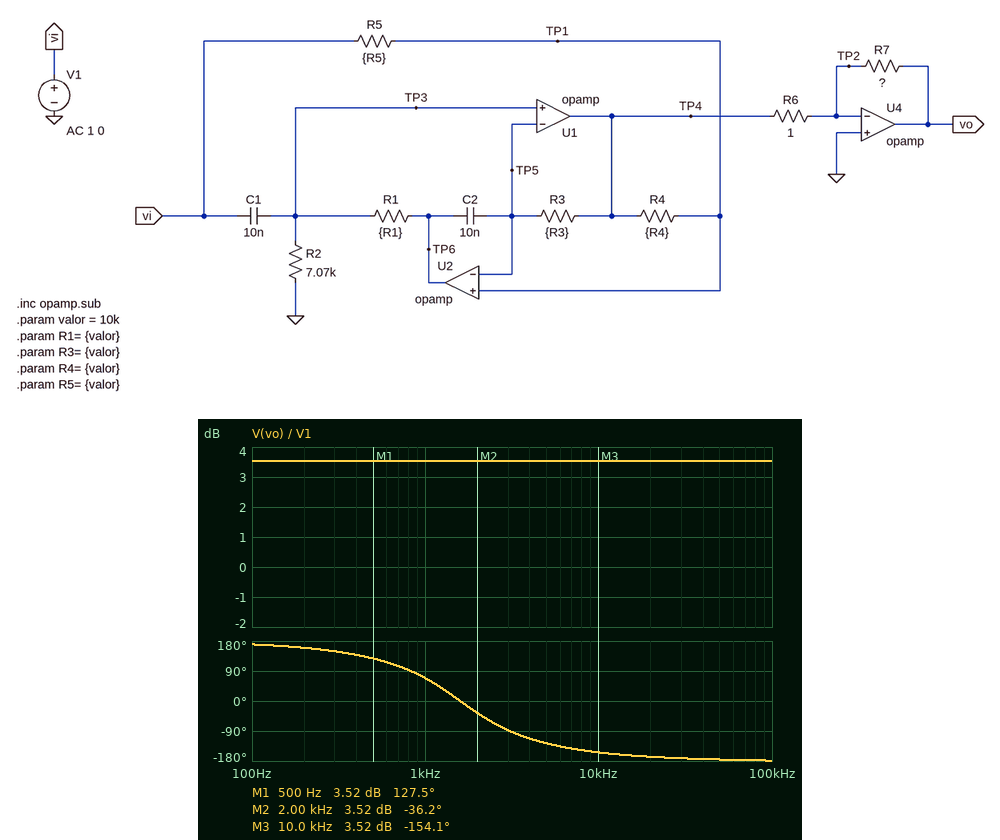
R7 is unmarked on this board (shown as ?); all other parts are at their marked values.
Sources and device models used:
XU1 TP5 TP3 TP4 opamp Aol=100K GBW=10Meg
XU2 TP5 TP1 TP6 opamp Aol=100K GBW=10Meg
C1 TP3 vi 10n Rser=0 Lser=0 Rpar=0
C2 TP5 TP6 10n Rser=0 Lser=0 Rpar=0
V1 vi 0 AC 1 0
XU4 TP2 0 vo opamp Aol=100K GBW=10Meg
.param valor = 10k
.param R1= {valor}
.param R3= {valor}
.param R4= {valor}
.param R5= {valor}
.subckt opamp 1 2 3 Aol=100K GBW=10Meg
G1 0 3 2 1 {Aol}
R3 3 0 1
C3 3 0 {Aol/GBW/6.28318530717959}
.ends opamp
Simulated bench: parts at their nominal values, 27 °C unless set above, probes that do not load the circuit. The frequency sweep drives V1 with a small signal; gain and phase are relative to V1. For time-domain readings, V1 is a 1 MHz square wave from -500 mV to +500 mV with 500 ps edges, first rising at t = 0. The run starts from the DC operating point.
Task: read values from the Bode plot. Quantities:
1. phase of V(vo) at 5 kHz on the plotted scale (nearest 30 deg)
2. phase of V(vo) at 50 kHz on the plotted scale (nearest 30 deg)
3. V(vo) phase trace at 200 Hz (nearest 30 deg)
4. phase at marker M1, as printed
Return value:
-120 deg
-180 deg
150 deg
127.5 deg
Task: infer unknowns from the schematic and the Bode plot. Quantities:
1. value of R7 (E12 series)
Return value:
1.5 Ω
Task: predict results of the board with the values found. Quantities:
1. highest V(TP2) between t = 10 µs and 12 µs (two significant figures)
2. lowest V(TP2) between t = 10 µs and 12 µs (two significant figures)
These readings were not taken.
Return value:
420 mV
-420 mV
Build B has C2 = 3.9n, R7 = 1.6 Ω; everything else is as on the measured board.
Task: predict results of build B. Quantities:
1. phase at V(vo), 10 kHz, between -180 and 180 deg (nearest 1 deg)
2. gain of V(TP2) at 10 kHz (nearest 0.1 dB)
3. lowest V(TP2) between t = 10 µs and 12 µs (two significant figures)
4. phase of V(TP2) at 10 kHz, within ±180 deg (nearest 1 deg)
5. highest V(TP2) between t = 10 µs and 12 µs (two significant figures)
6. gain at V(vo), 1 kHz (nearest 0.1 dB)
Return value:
-153 deg
-55.9 dB
-440 mV
116 deg
440 mV
4.1 dB
